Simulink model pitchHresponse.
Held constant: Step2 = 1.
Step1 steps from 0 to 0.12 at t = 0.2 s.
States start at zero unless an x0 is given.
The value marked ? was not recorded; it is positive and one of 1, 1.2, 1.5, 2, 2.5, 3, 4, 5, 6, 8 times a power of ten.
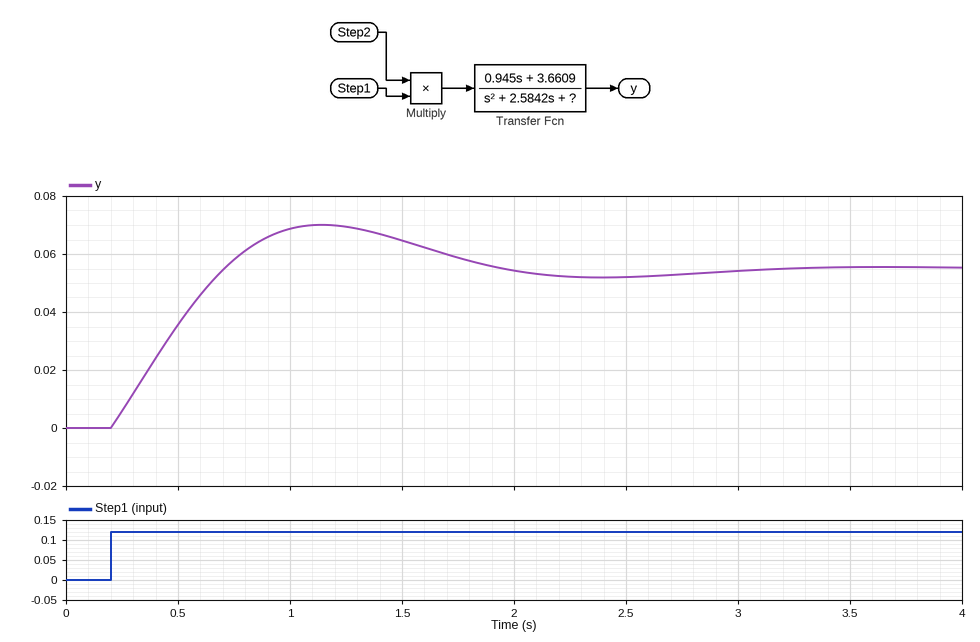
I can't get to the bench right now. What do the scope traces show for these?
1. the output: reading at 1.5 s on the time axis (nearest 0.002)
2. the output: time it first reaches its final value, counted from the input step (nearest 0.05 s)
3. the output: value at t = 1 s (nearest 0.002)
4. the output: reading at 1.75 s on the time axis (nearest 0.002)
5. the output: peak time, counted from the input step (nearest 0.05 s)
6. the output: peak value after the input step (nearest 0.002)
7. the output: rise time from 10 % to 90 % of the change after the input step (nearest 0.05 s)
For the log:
0.064
0.50 s
0.068
0.058
0.95 s
0.070
0.40 s
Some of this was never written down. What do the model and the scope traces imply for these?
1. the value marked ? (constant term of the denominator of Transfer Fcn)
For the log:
8
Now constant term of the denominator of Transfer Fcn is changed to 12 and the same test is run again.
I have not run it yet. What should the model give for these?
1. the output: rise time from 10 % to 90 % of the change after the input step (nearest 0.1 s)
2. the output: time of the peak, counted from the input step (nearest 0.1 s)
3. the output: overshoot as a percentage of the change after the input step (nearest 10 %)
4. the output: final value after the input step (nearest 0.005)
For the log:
0.3 s
0.7 s
40 %
0.035
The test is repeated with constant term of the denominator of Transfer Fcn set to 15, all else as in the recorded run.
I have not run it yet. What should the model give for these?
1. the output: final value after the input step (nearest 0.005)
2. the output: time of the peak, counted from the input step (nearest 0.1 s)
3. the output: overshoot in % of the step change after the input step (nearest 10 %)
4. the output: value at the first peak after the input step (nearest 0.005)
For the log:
0.030
0.6 s
50 %
0.045
